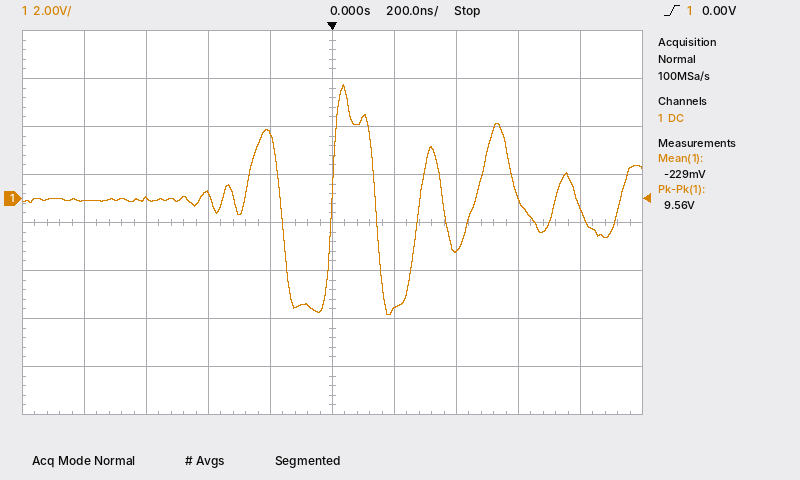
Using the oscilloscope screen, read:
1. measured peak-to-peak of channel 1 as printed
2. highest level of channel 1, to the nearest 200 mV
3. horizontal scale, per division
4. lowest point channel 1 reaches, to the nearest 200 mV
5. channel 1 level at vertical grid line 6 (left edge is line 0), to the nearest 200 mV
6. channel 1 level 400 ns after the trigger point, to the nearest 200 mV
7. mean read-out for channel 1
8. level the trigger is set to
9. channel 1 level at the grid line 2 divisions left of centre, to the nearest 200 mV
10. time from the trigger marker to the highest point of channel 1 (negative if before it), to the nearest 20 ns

9.56 V
4.8 V
200 ns
-4.8 V
-4.6 V
-2.2 V
-229 mV
0.00 V
200 mV
+40 ns
